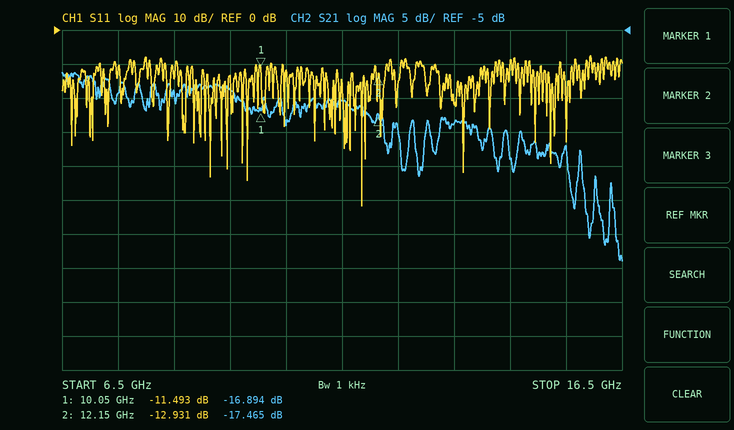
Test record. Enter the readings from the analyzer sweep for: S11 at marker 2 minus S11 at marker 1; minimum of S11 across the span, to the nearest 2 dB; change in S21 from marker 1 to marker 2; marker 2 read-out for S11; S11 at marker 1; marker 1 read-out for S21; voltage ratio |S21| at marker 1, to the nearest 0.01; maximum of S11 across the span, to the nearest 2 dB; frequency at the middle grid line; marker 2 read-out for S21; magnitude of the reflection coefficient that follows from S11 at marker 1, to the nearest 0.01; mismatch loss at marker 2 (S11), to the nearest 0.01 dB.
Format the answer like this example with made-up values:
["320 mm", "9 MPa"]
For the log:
["-1.438 dB", "-52 dB", "-0.571 dB", "-12.931 dB", "-11.493 dB", "-16.894 dB", "0.14", "-8 dB", "11.5 GHz", "-17.465 dB", "0.27", "0.23 dB"]
